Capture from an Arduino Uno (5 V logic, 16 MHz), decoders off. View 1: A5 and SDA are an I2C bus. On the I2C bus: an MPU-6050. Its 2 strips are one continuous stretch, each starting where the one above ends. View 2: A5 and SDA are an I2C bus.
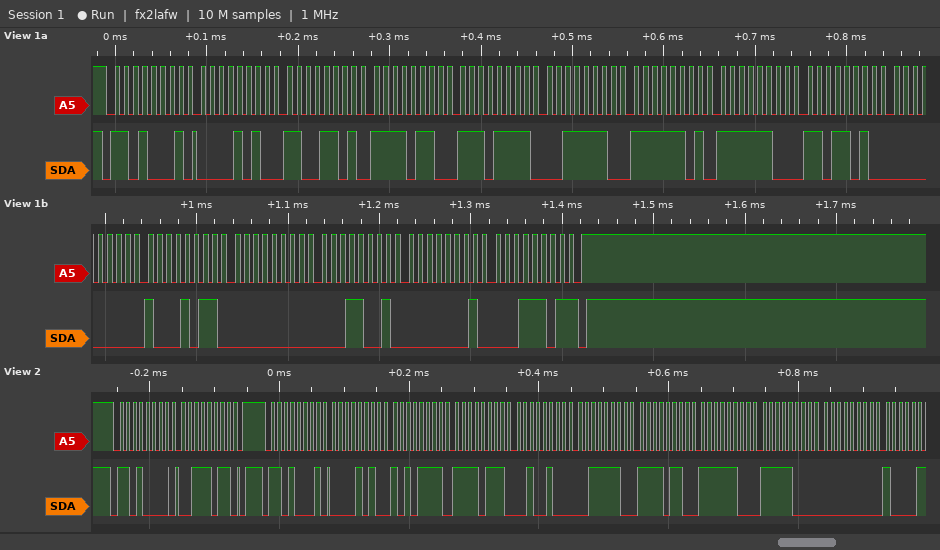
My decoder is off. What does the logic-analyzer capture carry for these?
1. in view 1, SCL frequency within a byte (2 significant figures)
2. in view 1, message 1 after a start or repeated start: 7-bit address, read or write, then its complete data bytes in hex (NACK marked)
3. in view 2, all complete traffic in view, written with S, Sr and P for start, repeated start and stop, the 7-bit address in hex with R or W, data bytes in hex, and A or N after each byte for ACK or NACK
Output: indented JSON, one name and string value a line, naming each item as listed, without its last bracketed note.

{
  "in view 1, SCL frequency within a byte": "100 kHz",
  "in view 1, message 1 after a start or repeated start: 7-bit address, read or write, then its complete data bytes in hex": "0x68 read: 0A CD F6 EF 3E FD FC DA 00 8B 00 19 01 1D NACK",
  "in view 2, all complete traffic in view, written with S, Sr and P for start, repeated start and stop, the 7-bit address in hex with R or W, data bytes in hex, and A or N after each byte for ACK or NACK": "S 68W A 3B A P S 68R A 0A A AF A F7 A 24 A 3E A F6 A FC A F8 A 00 A"
}
